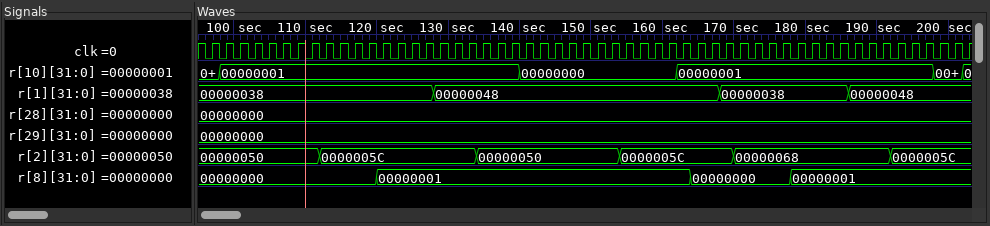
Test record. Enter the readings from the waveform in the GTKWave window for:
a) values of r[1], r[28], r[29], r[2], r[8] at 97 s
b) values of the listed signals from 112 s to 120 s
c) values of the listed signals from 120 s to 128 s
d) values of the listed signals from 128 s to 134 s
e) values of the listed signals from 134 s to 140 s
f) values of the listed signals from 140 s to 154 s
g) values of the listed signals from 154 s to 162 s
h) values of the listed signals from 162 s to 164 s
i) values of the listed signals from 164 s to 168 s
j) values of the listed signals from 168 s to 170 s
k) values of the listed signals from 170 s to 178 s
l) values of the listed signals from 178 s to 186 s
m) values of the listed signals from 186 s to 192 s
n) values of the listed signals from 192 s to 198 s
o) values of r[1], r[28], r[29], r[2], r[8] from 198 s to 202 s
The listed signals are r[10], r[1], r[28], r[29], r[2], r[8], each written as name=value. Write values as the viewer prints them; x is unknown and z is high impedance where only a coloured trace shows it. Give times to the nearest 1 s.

r[1]=00000038, r[28]=00000000, r[29]=00000000, r[2]=00000050, r[8]=00000000
r[10]=00000001, r[1]=00000038, r[28]=00000000, r[29]=00000000, r[2]=0000005C, r[8]=00000000
r[10]=00000001, r[1]=00000038, r[28]=00000000, r[29]=00000000, r[2]=0000005C, r[8]=00000001
r[10]=00000001, r[1]=00000048, r[28]=00000000, r[29]=00000000, r[2]=0000005C, r[8]=00000001
r[10]=00000001, r[1]=00000048, r[28]=00000000, r[29]=00000000, r[2]=00000050, r[8]=00000001
r[10]=00000000, r[1]=00000048, r[28]=00000000, r[29]=00000000, r[2]=00000050, r[8]=00000001
r[10]=00000000, r[1]=00000048, r[28]=00000000, r[29]=00000000, r[2]=0000005C, r[8]=00000001
r[10]=00000001, r[1]=00000048, r[28]=00000000, r[29]=00000000, r[2]=0000005C, r[8]=00000001
r[10]=00000001, r[1]=00000048, r[28]=00000000, r[29]=00000000, r[2]=0000005C, r[8]=00000000
r[10]=00000001, r[1]=00000038, r[28]=00000000, r[29]=00000000, r[2]=0000005C, r[8]=00000000
r[10]=00000001, r[1]=00000038, r[28]=00000000, r[29]=00000000, r[2]=00000068, r[8]=00000000
r[10]=00000001, r[1]=00000038, r[28]=00000000, r[29]=00000000, r[2]=00000068, r[8]=00000001
r[10]=00000001, r[1]=00000048, r[28]=00000000, r[29]=00000000, r[2]=00000068, r[8]=00000001
r[10]=00000001, r[1]=00000048, r[28]=00000000, r[29]=00000000, r[2]=0000005C, r[8]=00000001
r[1]=00000048, r[28]=00000000, r[29]=00000000, r[2]=0000005C, r[8]=00000001
